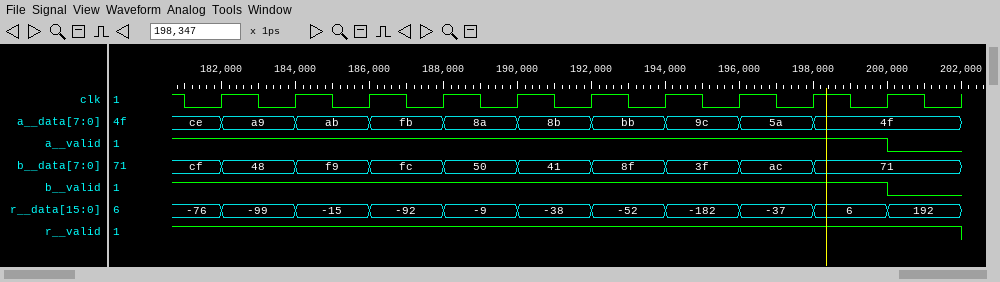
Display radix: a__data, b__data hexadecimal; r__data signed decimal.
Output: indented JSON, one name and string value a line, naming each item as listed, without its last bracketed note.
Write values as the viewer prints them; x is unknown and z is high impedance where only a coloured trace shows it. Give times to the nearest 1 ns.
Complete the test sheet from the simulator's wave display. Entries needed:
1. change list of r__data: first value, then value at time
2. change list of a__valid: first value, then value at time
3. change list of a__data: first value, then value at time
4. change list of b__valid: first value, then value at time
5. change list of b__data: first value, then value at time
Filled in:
{
  "change list of r__data: first value, then value at time": "-76, -99 at 182 ns, -15 at 184 ns, -92 at 186 ns, -9 at 188 ns, -38 at 190 ns, -52 at 192 ns, -182 at 194 ns, -37 at 196 ns, 6 at 198 ns, 192 at 200 ns",
  "change list of a__valid: first value, then value at time": "1, 0 at 200 ns",
  "change list of a__data: first value, then value at time": "ce, a9 at 182 ns, ab at 184 ns, fb at 186 ns, 8a at 188 ns, 8b at 190 ns, bb at 192 ns, 9c at 194 ns, 5a at 196 ns, 4f at 198 ns",
  "change list of b__valid: first value, then value at time": "1, 0 at 200 ns",
  "change list of b__data: first value, then value at time": "cf, 48 at 182 ns, f9 at 184 ns, fc at 186 ns, 50 at 188 ns, 41 at 190 ns, 8f at 192 ns, 3f at 194 ns, ac at 196 ns, 71 at 198 ns"
}
